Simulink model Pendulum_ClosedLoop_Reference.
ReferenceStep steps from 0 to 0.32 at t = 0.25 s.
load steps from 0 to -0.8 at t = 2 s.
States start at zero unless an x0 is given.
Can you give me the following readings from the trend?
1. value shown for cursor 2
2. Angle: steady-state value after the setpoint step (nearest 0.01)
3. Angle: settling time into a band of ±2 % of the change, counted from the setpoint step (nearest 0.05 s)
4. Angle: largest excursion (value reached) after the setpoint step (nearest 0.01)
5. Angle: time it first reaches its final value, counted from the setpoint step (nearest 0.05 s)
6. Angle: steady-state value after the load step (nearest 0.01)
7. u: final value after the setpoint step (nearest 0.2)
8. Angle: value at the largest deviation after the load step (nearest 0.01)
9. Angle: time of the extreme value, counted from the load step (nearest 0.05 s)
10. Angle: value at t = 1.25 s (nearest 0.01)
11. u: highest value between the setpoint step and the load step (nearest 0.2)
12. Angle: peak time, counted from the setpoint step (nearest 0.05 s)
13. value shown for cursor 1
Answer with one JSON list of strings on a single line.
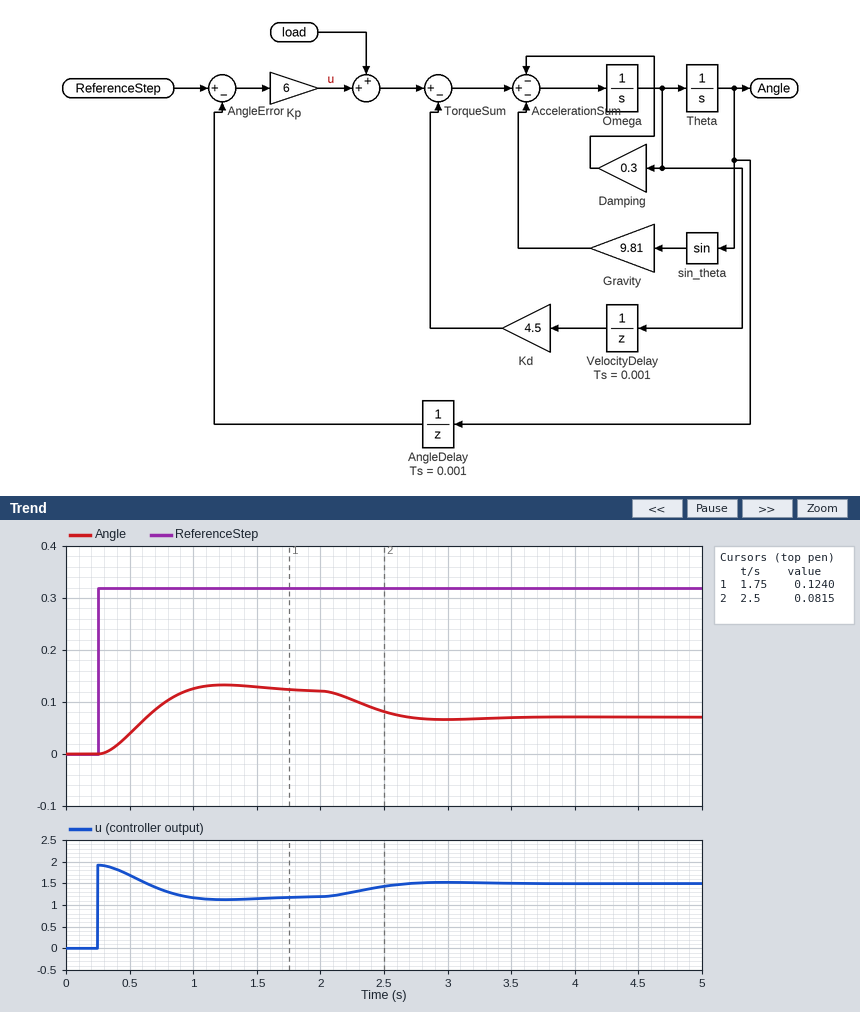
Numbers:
["0.0815", "0.12", "1.50 s", "0.13", "0.70 s", "0.07", "1.2", "0.07", "1.00 s", "0.13", "2.0", "1.00 s", "0.1240"]
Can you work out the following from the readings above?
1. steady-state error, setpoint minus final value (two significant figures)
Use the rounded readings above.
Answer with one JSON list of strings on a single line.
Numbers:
["0.20"]
